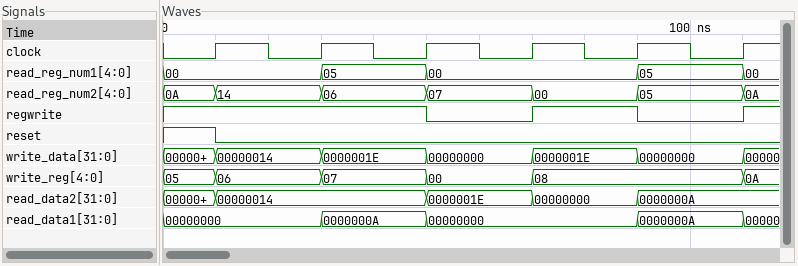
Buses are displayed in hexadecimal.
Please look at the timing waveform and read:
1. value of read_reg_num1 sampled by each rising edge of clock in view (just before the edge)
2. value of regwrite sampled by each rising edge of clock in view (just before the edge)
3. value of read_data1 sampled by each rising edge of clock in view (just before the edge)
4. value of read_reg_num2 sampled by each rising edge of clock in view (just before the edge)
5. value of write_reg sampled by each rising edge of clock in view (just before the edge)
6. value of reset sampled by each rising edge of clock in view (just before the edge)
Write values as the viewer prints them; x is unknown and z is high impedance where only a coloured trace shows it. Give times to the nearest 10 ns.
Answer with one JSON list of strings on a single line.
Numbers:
["00, 00, 05, 00, 00, 05", "1 1 1 0 1 0", "00000000, 00000000, 0000000A, 00000000, 00000000, 0000000A", "0A, 14, 06, 07, 00, 05", "05, 06, 07, 00, 08, 08", "1 0 0 0 0 0"]
